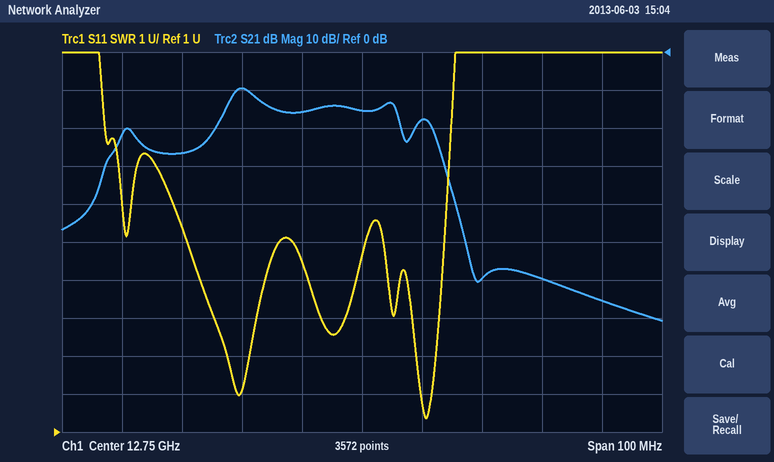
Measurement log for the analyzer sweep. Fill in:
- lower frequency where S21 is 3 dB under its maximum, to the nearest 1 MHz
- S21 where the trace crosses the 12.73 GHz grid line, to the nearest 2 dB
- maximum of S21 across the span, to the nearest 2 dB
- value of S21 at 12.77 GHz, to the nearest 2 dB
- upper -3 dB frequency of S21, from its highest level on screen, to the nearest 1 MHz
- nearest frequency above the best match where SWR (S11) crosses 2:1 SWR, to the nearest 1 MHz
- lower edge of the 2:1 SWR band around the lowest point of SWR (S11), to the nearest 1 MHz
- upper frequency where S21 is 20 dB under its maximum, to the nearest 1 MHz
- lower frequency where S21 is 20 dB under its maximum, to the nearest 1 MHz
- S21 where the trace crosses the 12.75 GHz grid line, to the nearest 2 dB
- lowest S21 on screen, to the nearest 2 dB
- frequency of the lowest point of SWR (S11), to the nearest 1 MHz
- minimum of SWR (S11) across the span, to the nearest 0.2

12.728 GHz
-10 dB
-10 dB
-60 dB
12.733 GHz
12.762 GHz
12.760 GHz
12.764 GHz
12.707 GHz
-16 dB
-70 dB
12.761 GHz
1.4
